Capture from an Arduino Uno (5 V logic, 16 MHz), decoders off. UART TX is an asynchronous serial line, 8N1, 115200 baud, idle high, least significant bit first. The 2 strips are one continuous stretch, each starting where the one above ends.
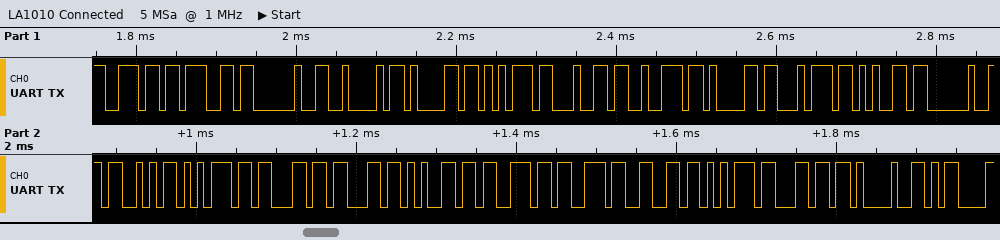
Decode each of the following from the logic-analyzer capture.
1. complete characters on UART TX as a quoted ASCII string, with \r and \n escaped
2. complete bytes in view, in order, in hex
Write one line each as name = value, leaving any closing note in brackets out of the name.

complete characters on UART TX as a quoted ASCII string, with \r and \n escaped = "ng Baudrate Successful!\r"
complete bytes in view, in order, in hex = 6E 67 20 42 61 75 64 72 61 74 65 20 53 75 63 63 65 73 73 66 75 6C 21 0D
